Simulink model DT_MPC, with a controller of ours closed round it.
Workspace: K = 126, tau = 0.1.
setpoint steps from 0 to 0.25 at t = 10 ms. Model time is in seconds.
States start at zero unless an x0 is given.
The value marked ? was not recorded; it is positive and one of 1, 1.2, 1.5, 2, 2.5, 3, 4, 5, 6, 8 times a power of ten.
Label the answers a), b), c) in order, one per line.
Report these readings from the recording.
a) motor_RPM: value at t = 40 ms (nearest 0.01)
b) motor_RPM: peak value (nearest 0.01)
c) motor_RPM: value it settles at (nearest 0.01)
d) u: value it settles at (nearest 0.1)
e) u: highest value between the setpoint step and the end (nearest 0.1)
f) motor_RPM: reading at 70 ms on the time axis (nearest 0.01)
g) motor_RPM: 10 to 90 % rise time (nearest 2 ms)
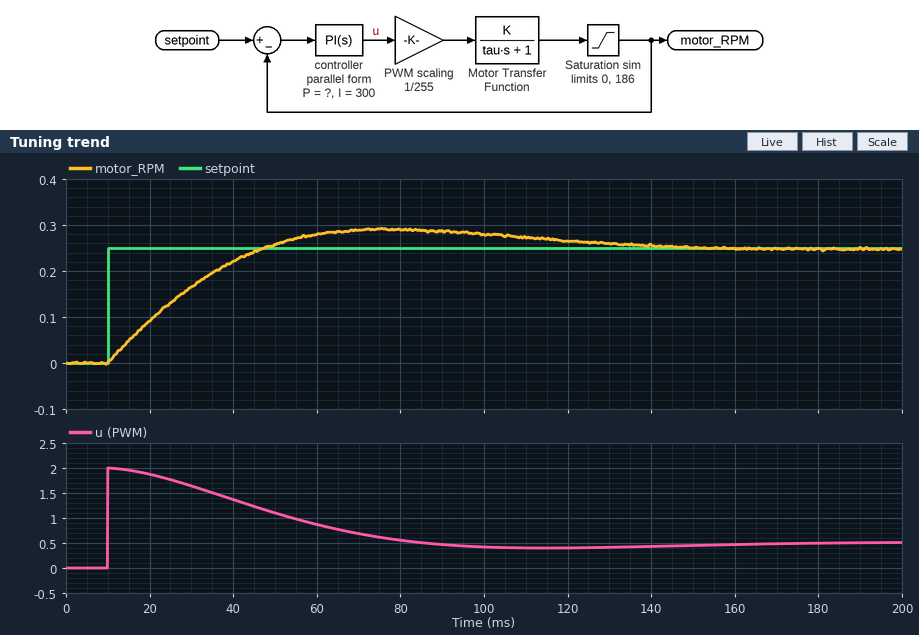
a) 0.22
b) 0.29
c) 0.25
d) 0.5
e) 2.0
f) 0.29
g) 28 ms
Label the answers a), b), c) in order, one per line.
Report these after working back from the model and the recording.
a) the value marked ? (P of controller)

a) 8
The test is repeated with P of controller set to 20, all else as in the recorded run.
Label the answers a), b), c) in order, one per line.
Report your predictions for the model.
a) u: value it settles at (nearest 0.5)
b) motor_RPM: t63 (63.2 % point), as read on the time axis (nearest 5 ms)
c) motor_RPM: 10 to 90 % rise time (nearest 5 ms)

a) 0.5
b) 20 ms
c) 20 ms
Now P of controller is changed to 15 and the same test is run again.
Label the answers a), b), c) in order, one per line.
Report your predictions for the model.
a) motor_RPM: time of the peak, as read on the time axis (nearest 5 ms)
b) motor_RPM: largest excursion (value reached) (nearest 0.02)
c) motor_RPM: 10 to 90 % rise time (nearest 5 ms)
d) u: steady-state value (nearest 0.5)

a) 70 ms
b) 0.26
c) 25 ms
d) 0.5
